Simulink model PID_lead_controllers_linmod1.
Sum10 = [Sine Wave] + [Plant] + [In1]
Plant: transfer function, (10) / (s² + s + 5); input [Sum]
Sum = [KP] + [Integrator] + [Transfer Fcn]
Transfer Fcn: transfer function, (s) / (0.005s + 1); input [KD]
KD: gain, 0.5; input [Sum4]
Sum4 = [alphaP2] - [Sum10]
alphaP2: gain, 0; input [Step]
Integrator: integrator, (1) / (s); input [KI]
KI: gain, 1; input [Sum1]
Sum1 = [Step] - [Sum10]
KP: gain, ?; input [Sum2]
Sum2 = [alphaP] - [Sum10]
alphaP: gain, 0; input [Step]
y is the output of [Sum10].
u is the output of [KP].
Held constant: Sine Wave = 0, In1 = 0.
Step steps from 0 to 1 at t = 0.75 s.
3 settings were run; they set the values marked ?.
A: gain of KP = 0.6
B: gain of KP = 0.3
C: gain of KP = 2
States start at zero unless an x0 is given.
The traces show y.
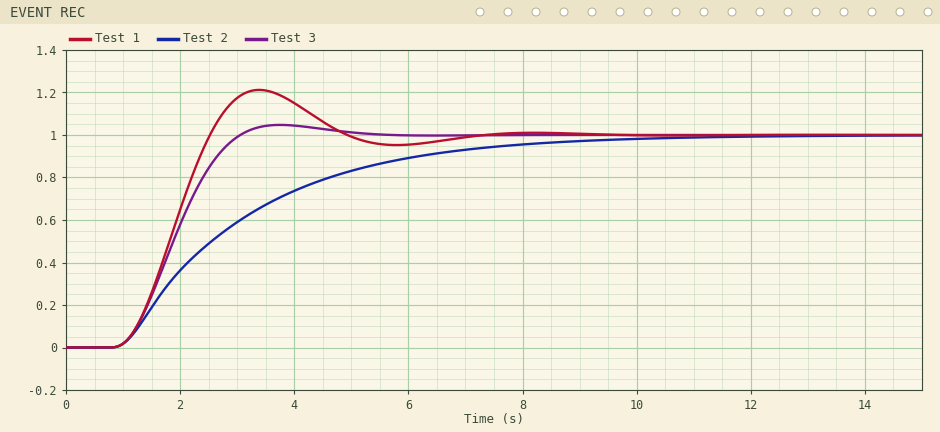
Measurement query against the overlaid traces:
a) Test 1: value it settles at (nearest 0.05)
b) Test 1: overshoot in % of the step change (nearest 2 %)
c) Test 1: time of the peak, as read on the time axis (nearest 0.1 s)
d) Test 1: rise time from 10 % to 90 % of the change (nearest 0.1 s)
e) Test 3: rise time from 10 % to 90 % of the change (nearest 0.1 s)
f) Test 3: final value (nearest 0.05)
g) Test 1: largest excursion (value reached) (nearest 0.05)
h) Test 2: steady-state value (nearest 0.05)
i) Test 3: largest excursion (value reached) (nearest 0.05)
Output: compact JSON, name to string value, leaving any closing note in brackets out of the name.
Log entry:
{"Test 1: value it settles at": "1.00", "Test 1: overshoot in % of the step change": "22 %", "Test 1: time of the peak, as read on the time axis": "3.4 s", "Test 1: rise time from 10 % to 90 % of the change": "1.1 s", "Test 3: rise time from 10 % to 90 % of the change": "1.4 s", "Test 3: final value": "1.00", "Test 1: largest excursion (value reached)": "1.20", "Test 2: steady-state value": "1.00", "Test 3: largest excursion (value reached)": "1.05"}
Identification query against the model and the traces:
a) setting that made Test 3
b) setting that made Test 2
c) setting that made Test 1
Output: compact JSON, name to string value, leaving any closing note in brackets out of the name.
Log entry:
{"setting that made Test 3": "A", "setting that made Test 2": "C", "setting that made Test 1": "B"}
